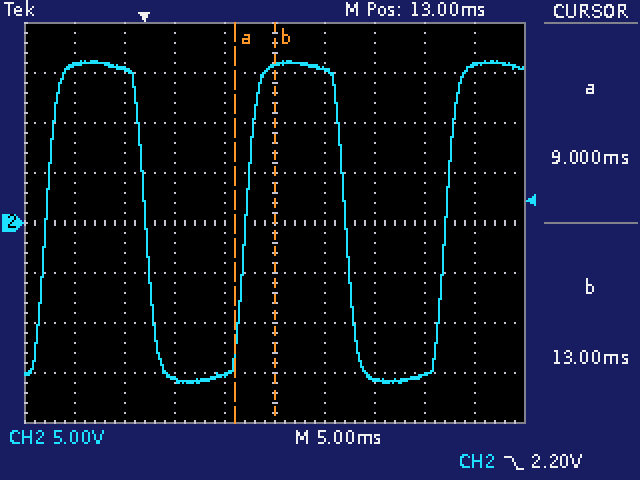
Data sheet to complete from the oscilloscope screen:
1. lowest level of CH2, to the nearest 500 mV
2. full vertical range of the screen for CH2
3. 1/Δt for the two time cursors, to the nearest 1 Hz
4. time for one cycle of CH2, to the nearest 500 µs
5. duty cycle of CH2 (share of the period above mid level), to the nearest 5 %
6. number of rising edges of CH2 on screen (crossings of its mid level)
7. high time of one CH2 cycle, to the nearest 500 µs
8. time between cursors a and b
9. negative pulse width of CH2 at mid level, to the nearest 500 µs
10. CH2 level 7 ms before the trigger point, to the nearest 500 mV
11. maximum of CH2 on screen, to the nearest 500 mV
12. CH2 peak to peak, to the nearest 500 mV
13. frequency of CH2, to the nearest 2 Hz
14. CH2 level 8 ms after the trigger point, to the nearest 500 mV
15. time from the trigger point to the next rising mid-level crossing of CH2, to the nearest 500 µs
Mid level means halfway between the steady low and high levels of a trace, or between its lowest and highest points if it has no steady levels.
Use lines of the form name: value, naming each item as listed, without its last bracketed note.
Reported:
lowest level of CH2, to the nearest 500 mV: -16.0 V
full vertical range of the screen for CH2: 40 V
1/Δt for the two time cursors, to the nearest 1 Hz: 250 Hz
time for one cycle of CH2, to the nearest 500 µs: 20.0 ms
duty cycle of CH2 (share of the period above mid level), to the nearest 5 %: 50 %
number of rising edges of CH2 on screen: 3
high time of one CH2 cycle, to the nearest 500 µs: 10.0 ms
time between cursors a and b: 4.0 ms
negative pulse width of CH2 at mid level, to the nearest 500 µs: 10.0 ms
CH2 level 7 ms before the trigger point, to the nearest 500 mV: 16.0 V
maximum of CH2 on screen, to the nearest 500 mV: 16.0 V
CH2 peak to peak, to the nearest 500 mV: 32.0 V
frequency of CH2, to the nearest 2 Hz: 50 Hz
CH2 level 8 ms after the trigger point, to the nearest 500 mV: -15.0 V
time from the trigger point to the next rising mid-level crossing of CH2, to the nearest 500 µs: 10.0 ms
